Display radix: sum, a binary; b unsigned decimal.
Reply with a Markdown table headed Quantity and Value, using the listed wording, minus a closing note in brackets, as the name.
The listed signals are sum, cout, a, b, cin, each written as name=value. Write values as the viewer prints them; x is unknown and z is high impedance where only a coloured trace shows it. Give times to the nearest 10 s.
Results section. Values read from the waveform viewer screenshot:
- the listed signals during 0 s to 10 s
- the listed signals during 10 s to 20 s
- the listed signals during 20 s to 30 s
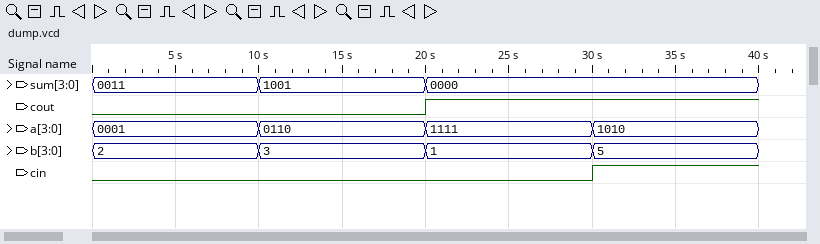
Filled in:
| Quantity | Value |
|---|---|
| the listed signals during 0 s to 10 s | sum=0011, cout=0, a=0001, b=2, cin=0 |
| the listed signals during 10 s to 20 s | sum=1001, cout=0, a=0110, b=3, cin=0 |
| the listed signals during 20 s to 30 s | sum=0000, cout=1, a=1111, b=1, cin=0 |
